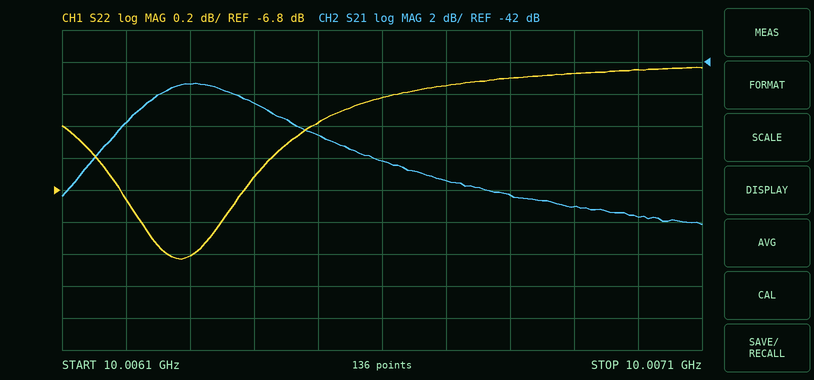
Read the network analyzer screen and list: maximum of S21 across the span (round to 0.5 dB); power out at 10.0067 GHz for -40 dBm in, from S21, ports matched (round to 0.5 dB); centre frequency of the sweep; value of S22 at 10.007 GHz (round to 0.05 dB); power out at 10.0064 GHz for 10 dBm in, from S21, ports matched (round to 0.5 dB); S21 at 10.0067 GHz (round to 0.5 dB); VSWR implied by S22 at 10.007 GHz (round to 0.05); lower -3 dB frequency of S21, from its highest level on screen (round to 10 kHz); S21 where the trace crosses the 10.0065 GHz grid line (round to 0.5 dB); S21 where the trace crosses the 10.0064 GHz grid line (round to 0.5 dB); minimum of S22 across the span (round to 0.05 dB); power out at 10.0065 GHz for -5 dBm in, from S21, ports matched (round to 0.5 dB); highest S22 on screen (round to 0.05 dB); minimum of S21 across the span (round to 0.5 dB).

-43.5 dB
-89.5 dBm
10.0066 GHz
-6.05 dB
-34.5 dBm
-49.5 dB
3.00
10.00619 GHz
-46.5 dB
-44.5 dB
-7.25 dB
-51.5 dBm
-6.05 dB
-52.0 dB
